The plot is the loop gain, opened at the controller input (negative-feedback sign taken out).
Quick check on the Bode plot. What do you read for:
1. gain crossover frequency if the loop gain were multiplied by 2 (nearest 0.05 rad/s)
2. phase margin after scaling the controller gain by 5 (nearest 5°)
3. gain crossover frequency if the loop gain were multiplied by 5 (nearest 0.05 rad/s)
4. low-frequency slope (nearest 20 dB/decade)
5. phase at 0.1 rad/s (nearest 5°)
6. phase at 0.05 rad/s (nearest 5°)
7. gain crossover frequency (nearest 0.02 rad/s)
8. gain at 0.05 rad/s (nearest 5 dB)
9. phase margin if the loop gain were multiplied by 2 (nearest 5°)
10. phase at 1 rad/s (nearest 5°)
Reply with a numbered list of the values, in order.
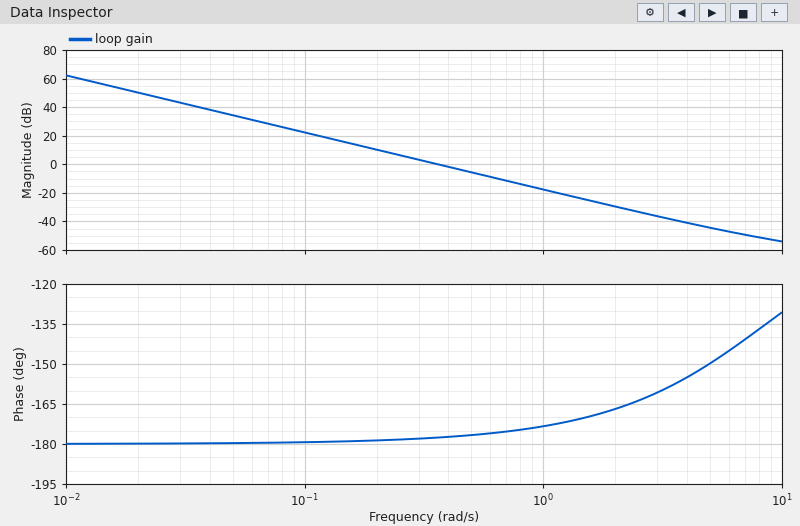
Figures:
1. 0.50 rad/s
2. 5°
3. 0.80 rad/s
4. -40 dB/decade
5. -180°
6. -180°
7. 0.36 rad/s
8. 35 dB
9. 5°
10. -175°
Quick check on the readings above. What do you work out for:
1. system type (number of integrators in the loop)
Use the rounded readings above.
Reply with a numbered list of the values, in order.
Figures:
1. 2
